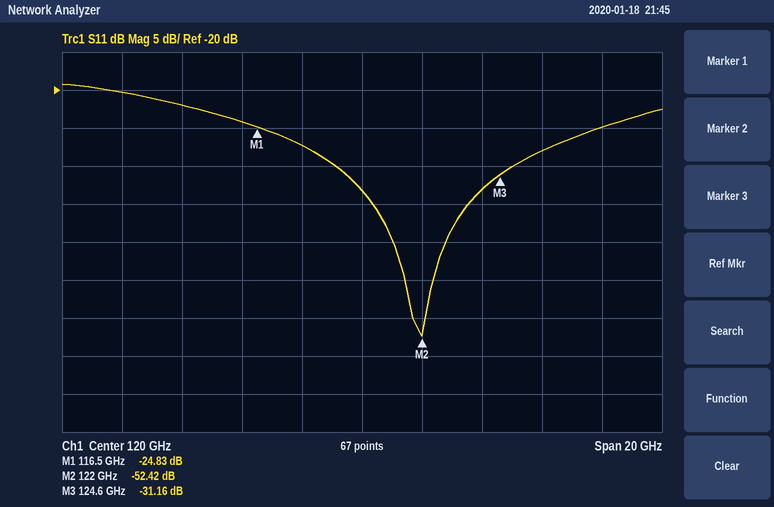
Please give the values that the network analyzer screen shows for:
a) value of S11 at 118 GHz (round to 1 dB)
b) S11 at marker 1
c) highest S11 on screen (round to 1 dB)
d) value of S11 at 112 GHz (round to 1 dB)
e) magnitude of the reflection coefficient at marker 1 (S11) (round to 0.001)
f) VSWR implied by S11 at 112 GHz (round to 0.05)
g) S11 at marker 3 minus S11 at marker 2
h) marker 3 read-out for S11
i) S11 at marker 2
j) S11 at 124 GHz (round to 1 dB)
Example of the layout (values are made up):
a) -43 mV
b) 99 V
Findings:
a) -27 dB
b) -24.83 dB
c) -19 dB
d) -20 dB
e) 0.057
f) 1.20
g) 21.26 dB
h) -31.16 dB
i) -52.42 dB
j) -33 dB
